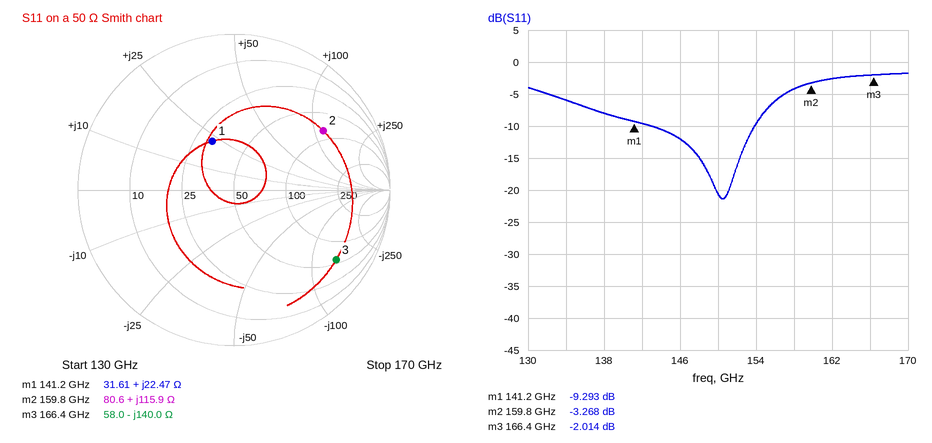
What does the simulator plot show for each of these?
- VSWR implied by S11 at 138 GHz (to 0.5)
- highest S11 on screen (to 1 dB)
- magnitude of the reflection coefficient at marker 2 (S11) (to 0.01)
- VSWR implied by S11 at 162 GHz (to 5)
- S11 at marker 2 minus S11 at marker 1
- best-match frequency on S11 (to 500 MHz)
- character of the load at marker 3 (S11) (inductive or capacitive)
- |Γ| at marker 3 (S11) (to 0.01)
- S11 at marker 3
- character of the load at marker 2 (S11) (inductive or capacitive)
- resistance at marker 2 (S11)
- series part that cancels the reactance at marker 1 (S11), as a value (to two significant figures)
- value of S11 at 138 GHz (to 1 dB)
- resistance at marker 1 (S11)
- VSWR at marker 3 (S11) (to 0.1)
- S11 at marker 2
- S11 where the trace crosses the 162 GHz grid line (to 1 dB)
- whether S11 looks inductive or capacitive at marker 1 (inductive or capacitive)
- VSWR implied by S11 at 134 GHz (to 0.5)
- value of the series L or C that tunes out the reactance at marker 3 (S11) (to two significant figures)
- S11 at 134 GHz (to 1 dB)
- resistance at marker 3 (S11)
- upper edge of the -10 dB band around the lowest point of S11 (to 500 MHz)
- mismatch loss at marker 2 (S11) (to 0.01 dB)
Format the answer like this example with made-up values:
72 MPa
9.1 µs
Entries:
2.5
-2 dB
0.69
5
6.025 dB
150.5 GHz
capacitive
0.79
-2.014 dB
inductive
80.6 Ω
50 fF
-8 dB
31.61 Ω
8.7
-3.268 dB
-3 dB
inductive
3.0
130 pH
-6 dB
58.0 Ω
154.0 GHz
2.77 dB
